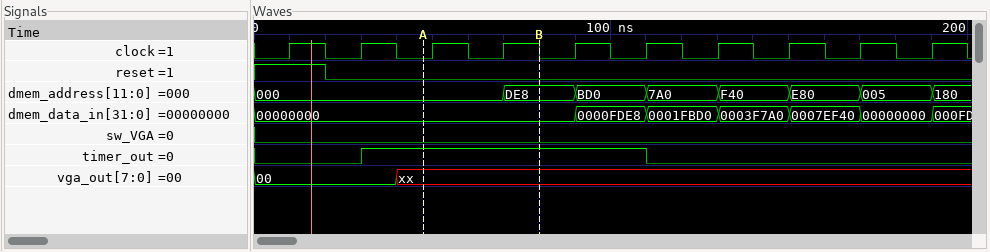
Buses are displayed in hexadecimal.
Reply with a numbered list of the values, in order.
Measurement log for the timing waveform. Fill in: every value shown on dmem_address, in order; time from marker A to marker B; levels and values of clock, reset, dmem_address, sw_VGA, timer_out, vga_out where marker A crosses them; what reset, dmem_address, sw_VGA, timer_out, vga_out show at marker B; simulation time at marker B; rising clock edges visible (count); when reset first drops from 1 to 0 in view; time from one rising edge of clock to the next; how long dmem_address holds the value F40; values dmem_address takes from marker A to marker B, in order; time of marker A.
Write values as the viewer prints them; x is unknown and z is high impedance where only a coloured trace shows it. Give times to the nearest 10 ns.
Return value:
1. 000, DE8, BD0, 7A0, F40, E80, 005, 180
2. 30 ns
3. clock=0, reset=0, dmem_address=000, sw_VGA=0, timer_out=1, vga_out=xx
4. reset=0, dmem_address=DE8, sw_VGA=0, timer_out=1, vga_out=xx
5. 80 ns
6. 10
7. 20 ns
8. 20 ns
9. 20 ns
10. 000, DE8
11. 50 ns
